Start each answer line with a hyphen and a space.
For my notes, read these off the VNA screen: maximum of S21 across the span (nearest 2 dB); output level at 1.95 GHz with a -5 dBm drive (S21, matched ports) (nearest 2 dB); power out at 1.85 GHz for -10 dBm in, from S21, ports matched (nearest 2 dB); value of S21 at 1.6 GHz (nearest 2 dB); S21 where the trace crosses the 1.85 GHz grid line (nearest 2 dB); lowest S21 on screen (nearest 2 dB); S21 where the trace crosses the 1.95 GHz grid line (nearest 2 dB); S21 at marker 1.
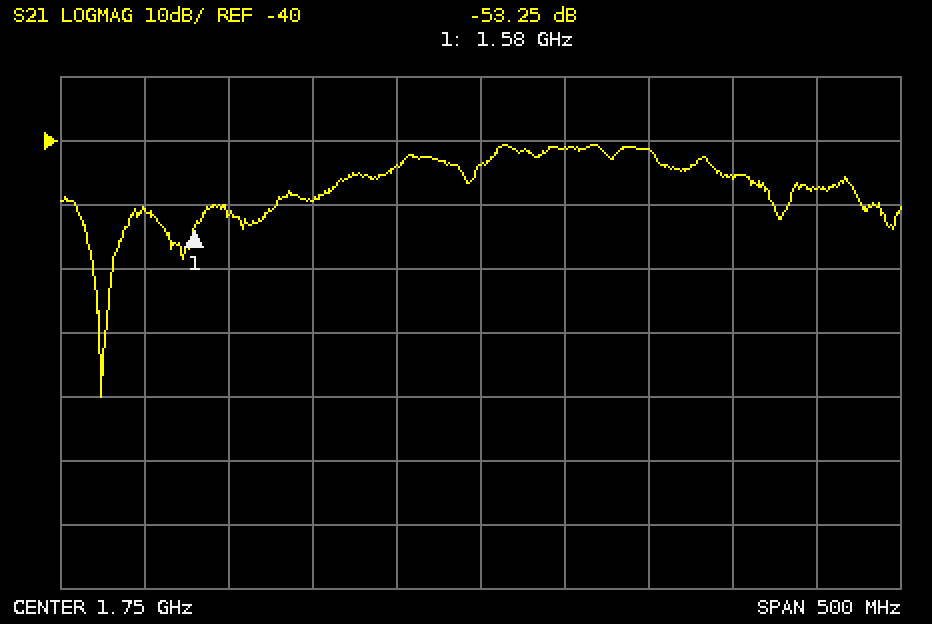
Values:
- -40 dB
- -52 dBm
- -52 dBm
- -52 dB
- -42 dB
- -80 dB
- -48 dB
- -53.25 dB
